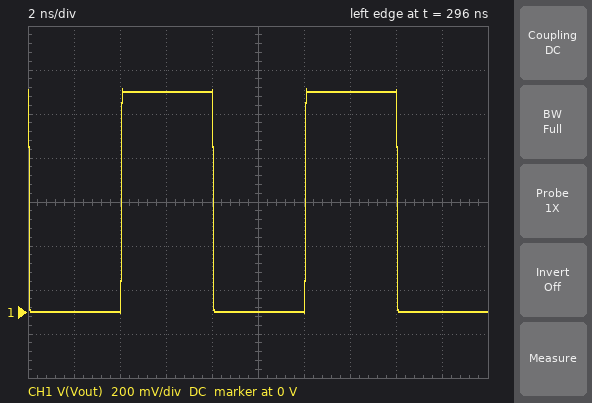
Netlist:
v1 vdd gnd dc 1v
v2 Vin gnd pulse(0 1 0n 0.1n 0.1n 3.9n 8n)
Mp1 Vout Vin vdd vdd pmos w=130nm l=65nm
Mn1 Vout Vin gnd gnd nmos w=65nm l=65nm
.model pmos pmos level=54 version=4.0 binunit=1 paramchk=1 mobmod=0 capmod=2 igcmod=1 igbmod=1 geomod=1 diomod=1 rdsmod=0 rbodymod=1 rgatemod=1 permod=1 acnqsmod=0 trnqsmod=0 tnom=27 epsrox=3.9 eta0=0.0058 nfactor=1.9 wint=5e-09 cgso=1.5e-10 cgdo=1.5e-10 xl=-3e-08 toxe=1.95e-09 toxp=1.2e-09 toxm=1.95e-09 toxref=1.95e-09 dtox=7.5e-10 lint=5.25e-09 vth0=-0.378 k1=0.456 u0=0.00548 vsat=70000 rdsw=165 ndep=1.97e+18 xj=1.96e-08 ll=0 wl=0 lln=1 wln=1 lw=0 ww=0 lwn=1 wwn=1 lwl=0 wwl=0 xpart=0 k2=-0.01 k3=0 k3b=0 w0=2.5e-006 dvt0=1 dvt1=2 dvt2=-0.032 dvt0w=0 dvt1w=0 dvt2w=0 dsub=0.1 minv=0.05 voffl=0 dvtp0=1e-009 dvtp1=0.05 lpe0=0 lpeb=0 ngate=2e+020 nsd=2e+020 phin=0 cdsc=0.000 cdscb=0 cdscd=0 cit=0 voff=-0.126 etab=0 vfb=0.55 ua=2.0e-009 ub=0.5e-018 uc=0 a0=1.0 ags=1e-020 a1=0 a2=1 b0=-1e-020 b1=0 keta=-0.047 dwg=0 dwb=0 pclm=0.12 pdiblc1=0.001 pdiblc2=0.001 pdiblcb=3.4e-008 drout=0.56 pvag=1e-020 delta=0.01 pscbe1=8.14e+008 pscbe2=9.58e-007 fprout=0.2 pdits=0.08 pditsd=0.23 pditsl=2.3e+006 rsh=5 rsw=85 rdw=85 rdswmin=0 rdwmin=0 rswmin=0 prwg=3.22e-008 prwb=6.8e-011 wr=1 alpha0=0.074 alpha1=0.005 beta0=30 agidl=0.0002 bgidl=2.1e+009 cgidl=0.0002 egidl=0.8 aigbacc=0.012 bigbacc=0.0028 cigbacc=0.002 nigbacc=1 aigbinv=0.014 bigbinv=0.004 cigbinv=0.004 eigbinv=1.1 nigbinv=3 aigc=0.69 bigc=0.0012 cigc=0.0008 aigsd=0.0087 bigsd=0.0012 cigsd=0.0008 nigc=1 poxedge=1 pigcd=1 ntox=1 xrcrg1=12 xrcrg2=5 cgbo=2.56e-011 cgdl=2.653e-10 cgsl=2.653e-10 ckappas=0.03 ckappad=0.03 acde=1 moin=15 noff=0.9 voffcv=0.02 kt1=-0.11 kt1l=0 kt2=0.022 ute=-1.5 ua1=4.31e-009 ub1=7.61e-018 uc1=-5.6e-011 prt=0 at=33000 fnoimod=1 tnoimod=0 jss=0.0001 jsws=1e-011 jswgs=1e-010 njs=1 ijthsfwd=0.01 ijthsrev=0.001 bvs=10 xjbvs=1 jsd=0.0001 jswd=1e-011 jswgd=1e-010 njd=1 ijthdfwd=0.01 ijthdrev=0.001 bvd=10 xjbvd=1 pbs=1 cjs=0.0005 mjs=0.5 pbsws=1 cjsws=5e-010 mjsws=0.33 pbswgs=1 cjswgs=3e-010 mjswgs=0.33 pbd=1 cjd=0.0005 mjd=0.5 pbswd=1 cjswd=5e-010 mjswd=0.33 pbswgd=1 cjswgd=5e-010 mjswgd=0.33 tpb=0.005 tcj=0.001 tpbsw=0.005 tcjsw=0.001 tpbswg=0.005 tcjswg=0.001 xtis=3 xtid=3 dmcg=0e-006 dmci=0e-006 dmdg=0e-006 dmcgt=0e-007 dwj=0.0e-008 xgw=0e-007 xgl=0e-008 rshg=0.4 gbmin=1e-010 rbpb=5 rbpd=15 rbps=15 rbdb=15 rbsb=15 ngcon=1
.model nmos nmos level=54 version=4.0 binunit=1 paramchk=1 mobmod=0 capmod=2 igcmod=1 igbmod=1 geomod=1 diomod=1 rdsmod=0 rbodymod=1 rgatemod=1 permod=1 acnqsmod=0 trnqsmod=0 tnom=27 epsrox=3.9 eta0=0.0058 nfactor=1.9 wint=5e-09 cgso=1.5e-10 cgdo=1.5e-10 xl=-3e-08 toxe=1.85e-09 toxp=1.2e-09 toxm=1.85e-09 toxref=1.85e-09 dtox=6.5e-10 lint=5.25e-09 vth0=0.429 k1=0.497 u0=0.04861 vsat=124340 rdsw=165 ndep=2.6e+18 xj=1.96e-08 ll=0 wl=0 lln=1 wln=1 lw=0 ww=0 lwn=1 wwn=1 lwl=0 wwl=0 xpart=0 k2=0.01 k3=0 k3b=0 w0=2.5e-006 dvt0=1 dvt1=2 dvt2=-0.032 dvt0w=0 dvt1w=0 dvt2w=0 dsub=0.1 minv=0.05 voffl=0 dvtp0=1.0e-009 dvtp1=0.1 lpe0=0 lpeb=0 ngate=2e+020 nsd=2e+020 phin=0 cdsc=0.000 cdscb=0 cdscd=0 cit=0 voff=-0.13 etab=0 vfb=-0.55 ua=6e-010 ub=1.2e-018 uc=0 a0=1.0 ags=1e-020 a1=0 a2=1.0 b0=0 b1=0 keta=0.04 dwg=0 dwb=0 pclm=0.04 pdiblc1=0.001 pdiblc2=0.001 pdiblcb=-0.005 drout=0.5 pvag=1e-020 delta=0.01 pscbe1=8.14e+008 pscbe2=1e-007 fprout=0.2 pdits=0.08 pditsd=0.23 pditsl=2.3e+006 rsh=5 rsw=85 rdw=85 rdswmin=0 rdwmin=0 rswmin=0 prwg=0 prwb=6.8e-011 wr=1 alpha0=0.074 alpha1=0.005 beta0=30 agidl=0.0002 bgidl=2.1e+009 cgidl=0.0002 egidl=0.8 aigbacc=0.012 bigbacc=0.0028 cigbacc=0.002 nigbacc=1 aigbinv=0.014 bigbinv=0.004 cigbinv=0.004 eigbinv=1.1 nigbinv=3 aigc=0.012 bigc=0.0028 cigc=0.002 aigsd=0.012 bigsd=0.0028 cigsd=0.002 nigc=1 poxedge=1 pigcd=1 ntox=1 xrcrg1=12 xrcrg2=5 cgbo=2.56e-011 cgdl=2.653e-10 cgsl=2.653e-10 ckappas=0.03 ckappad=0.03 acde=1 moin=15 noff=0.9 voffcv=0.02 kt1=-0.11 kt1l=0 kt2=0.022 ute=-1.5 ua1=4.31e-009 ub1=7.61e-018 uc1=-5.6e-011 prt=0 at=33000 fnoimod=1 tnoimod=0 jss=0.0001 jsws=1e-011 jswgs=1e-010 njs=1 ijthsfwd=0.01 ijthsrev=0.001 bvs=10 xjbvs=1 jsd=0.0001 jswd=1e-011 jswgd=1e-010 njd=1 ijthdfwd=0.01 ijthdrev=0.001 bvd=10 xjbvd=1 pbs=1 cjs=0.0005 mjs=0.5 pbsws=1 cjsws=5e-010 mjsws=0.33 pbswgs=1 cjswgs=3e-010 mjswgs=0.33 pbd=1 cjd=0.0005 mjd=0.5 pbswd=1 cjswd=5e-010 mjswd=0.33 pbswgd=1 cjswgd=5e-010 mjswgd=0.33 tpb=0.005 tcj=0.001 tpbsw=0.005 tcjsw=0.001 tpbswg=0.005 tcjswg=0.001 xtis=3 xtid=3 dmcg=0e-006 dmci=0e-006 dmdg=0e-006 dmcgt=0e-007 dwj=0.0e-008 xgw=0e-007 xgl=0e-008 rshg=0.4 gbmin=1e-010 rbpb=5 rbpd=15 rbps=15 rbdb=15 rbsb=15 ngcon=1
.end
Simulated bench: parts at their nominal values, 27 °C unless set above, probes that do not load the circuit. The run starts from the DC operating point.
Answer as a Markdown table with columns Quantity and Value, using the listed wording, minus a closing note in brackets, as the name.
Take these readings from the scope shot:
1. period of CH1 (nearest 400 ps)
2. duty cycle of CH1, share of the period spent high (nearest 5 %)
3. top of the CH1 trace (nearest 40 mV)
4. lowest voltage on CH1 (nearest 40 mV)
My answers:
| Quantity | Value |
|---|---|
| period of CH1 | 8.0 ns |
| duty cycle of CH1, share of the period spent high | 50 % |
| top of the CH1 trace | 1.00 V |
| lowest voltage on CH1 | 0 V |
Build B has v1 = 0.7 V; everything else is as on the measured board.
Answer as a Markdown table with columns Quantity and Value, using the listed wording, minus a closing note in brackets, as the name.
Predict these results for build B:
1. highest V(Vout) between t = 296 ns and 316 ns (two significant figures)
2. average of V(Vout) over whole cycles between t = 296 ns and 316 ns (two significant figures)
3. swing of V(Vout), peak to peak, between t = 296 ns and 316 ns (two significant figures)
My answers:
| Quantity | Value |
|---|---|
| highest V(Vout) between t = 296 ns and 316 ns | 720 mV |
| average of V(Vout) over whole cycles between t = 296 ns and 316 ns | 350 mV |
| swing of V(Vout), peak to peak, between t = 296 ns and 316 ns | 730 mV |
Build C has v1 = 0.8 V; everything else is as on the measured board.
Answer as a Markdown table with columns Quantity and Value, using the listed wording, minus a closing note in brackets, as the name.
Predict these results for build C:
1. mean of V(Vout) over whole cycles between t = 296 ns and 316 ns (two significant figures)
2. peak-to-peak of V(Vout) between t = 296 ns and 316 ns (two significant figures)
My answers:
| Quantity | Value |
|---|---|
| mean of V(Vout) over whole cycles between t = 296 ns and 316 ns | 400 mV |
| peak-to-peak of V(Vout) between t = 296 ns and 316 ns | 820 mV |
